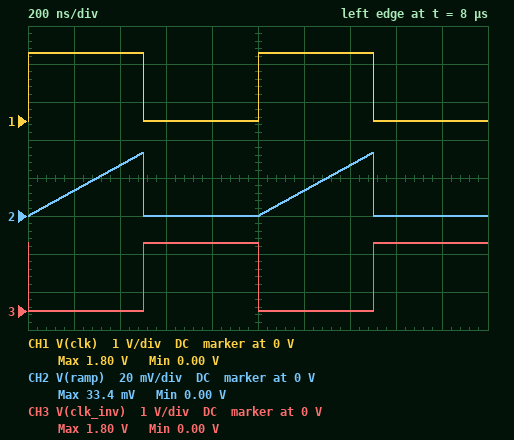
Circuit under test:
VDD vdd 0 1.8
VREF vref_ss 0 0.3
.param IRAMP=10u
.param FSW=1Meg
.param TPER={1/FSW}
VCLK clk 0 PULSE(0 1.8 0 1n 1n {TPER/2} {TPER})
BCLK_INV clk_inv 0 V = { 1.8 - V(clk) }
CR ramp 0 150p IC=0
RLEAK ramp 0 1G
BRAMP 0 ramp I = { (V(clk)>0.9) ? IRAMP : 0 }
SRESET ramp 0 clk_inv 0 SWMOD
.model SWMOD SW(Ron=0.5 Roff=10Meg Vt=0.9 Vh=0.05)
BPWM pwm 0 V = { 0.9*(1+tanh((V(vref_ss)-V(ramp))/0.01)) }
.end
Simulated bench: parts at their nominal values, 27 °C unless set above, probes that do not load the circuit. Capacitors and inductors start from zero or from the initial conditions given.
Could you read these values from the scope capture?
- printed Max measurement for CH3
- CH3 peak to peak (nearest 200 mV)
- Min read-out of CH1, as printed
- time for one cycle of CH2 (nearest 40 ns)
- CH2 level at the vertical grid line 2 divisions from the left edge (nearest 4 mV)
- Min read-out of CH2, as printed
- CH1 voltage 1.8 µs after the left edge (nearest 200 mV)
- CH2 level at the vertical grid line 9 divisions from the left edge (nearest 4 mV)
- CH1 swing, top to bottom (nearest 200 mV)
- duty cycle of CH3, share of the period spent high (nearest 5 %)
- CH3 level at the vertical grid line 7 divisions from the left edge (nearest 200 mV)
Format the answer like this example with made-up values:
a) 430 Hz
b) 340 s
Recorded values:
a) 1.80 V
b) 1.8 V
c) 0.00 V
d) 1.00 µs
e) 28 mV
f) 0.00 V
g) 0 V
h) 0 V
i) 1.8 V
j) 50 %
k) 0 V
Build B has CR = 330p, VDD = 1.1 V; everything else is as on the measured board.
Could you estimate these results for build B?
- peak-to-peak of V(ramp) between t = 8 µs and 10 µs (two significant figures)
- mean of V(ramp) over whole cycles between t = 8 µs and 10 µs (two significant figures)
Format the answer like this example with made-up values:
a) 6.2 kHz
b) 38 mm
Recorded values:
a) 15 mV
b) 3.8 mV
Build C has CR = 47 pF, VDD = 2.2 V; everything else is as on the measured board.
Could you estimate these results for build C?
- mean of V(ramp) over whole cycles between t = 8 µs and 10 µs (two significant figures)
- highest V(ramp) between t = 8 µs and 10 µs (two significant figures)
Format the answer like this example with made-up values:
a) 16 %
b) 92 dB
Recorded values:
a) 27 mV
b) 110 mV
